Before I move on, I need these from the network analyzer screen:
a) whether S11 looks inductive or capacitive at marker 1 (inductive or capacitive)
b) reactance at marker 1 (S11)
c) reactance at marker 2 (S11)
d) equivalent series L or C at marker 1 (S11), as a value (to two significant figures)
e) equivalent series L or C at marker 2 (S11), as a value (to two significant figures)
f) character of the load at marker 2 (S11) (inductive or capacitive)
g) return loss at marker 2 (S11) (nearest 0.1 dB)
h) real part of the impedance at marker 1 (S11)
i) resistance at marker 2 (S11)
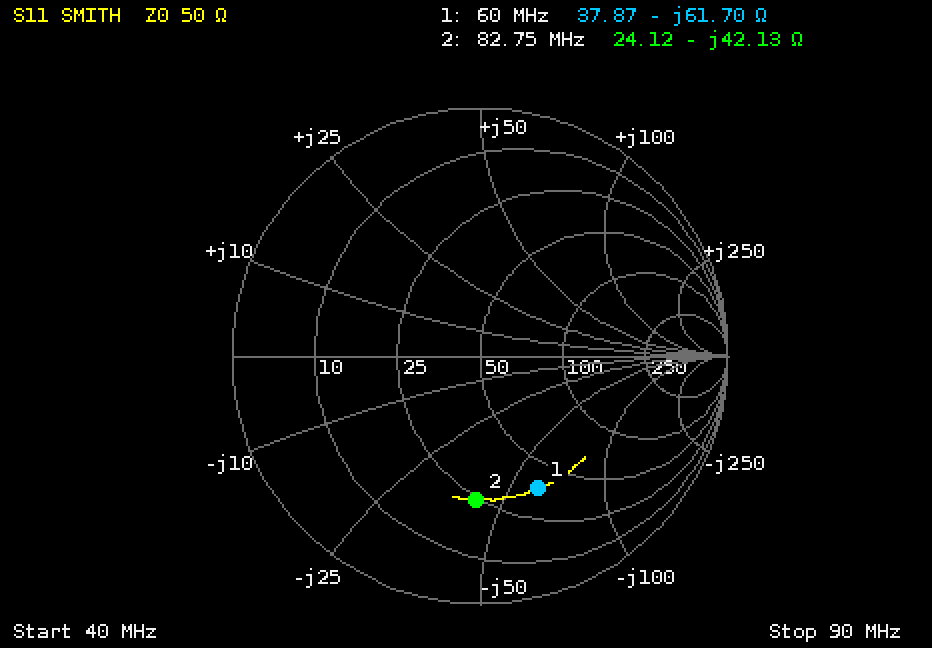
capacitive
-61.70 Ω
-42.13 Ω
43 pF
46 pF
capacitive
4.7 dB
37.87 Ω
24.12 Ω
